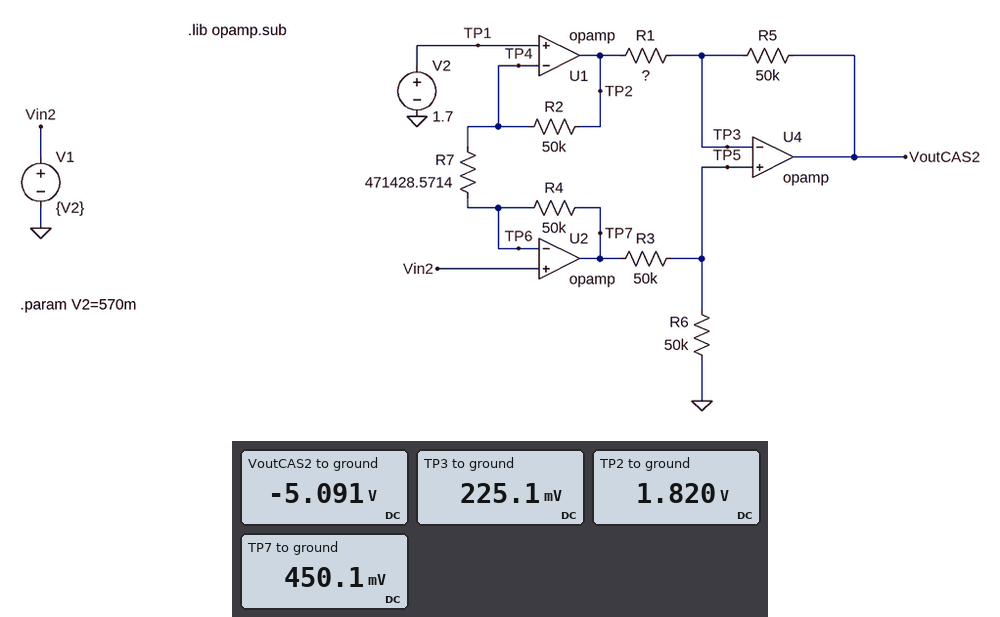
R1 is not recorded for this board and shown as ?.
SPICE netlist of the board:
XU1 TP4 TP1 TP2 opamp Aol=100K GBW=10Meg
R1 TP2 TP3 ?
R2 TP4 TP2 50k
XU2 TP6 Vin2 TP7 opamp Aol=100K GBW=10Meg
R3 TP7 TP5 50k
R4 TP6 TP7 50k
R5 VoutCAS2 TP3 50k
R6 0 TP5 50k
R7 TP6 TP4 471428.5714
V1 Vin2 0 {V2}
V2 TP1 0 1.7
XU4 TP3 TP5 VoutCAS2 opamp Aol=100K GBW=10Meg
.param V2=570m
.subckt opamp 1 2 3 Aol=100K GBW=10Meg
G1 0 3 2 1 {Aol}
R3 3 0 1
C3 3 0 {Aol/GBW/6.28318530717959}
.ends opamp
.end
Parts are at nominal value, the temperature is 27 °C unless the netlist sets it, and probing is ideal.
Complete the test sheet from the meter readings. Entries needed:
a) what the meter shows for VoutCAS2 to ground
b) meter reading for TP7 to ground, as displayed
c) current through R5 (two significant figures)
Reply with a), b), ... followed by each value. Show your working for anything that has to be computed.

a) -5.091 V
b) 450.1 mV
c) (225.1 mV - (-5.091 V)) / 50 kΩ = 110 µA
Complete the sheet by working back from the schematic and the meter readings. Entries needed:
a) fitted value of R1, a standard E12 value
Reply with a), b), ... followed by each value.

a) 15 kΩ
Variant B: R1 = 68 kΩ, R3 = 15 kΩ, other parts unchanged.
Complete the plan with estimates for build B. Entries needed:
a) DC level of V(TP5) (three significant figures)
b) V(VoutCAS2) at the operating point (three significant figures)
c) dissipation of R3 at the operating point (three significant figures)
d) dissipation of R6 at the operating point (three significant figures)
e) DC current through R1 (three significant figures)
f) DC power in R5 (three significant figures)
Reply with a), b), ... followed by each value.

a) 346 mV
b) -737 mV
c) 719 nW
d) 2.40 µW
e) 21.7 µA
f) 23.5 µW
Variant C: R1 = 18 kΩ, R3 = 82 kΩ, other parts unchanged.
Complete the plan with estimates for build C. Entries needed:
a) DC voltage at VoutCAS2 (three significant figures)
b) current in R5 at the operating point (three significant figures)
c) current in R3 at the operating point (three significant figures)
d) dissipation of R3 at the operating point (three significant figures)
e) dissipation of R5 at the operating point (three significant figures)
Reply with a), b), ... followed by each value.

a) -4.41 V
b) 91.6 µA
c) 3.41 µA
d) 954 nW
e) 420 µW
